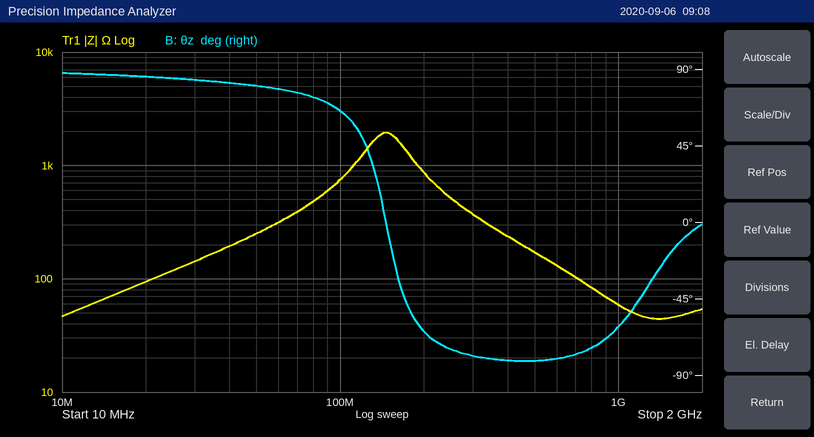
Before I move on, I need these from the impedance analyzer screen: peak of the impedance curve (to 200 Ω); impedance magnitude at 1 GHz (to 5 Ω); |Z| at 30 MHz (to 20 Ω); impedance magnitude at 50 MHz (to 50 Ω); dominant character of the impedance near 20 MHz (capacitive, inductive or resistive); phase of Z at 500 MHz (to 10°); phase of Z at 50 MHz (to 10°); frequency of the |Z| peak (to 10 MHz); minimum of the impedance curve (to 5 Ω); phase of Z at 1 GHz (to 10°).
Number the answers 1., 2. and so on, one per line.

1. 2.0 kΩ
2. 60 Ω
3. 140 Ω
4. 250 Ω
5. inductive
6. -80°
7. 80°
8. 150 MHz
9. 45 Ω
10. -60°
